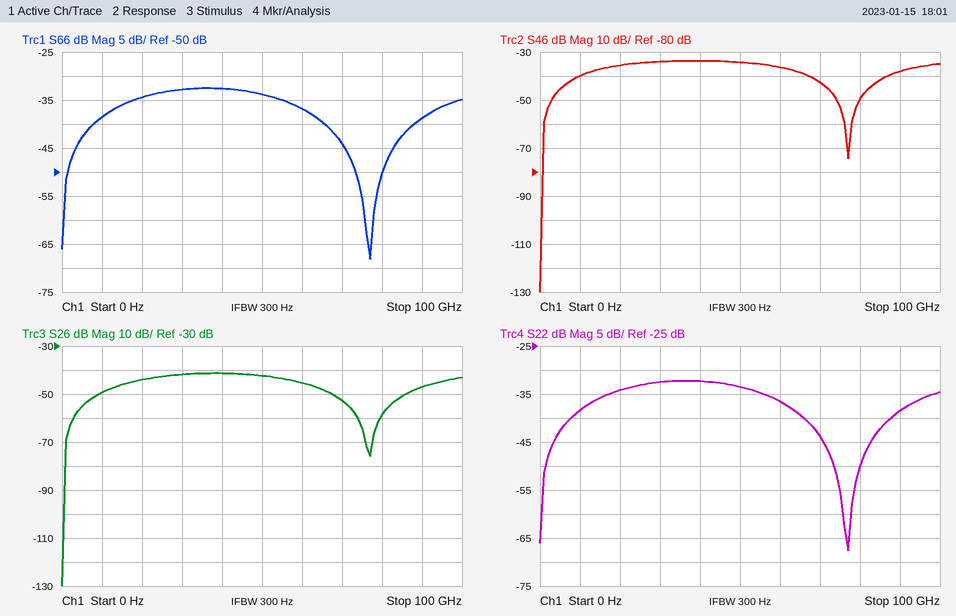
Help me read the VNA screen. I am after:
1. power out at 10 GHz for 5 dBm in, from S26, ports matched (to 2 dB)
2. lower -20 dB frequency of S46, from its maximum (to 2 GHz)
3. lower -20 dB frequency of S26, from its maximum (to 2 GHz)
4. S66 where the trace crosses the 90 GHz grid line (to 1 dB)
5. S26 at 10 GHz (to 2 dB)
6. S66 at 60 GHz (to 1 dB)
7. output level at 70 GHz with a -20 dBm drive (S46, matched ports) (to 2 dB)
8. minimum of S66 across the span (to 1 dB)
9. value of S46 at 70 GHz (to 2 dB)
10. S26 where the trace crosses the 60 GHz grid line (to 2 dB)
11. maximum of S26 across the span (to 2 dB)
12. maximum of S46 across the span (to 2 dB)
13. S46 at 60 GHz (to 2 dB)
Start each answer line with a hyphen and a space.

- -44 dBm
- 2 GHz
- 2 GHz
- -39 dB
- -50 dB
- -37 dB
- -62 dBm
- -68 dB
- -42 dB
- -46 dB
- -42 dB
- -34 dB
- -36 dB
